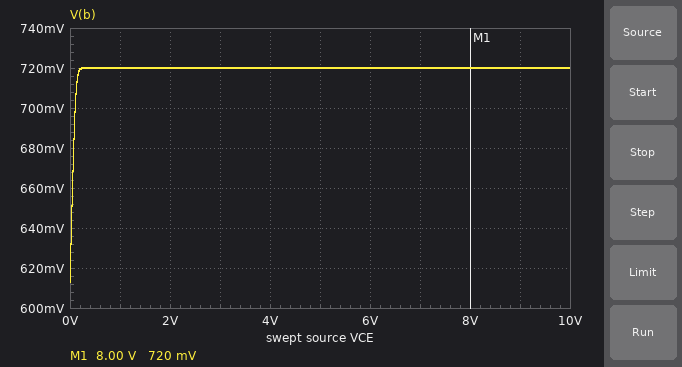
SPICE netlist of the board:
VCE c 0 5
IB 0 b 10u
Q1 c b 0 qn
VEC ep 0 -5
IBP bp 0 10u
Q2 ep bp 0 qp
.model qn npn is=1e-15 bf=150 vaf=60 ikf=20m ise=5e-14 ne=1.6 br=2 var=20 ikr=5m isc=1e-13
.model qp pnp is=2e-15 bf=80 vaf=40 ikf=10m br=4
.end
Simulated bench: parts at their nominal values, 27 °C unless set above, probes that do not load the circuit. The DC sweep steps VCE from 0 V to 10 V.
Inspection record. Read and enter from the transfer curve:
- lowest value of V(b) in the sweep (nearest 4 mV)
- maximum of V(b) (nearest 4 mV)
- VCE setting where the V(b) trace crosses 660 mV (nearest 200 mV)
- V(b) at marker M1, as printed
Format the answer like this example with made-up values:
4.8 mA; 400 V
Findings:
612 mV; 720 mV; 0 V; 720 mV
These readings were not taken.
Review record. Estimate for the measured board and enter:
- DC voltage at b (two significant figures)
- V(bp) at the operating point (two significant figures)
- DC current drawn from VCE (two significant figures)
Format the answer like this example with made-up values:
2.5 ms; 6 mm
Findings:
720 mV; -690 mV; 1.2 mA
